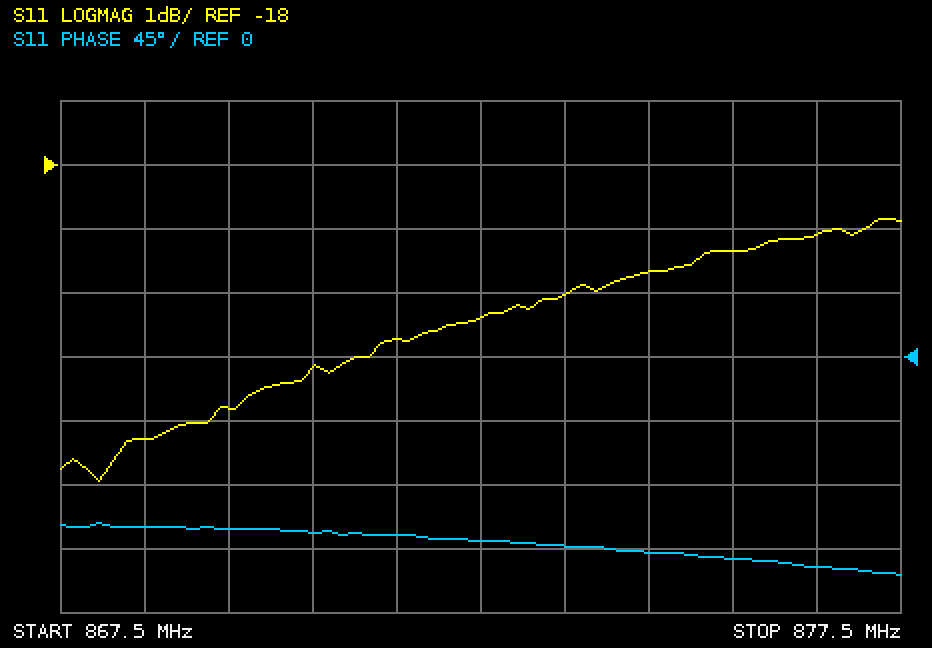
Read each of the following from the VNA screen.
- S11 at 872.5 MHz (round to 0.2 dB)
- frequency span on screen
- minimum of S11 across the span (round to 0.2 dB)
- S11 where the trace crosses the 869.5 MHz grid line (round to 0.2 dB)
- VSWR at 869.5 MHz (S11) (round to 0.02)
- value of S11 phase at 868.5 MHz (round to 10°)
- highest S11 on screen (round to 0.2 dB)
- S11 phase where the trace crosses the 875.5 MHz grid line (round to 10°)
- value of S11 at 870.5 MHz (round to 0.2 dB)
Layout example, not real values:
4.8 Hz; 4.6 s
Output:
-20.4 dB; 10 MHz; -23.0 dB; -21.8 dB; 1.18; -120°; -18.8 dB; -140°; -21.2 dB
